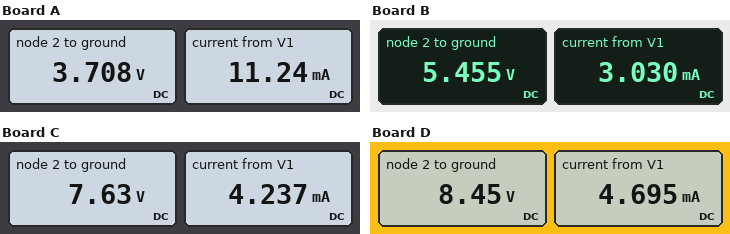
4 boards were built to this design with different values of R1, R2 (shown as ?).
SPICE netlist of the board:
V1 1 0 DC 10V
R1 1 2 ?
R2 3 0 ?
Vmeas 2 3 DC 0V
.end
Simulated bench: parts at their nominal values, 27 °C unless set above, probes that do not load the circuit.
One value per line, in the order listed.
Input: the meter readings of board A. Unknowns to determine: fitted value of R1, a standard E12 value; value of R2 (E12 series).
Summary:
560 Ω
330 Ω
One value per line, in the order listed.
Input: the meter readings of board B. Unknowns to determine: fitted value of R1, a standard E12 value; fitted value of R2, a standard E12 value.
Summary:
1.5 kΩ
1.8 kΩ
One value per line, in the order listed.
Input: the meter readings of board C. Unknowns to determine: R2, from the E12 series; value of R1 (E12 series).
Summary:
1.8 kΩ
560 Ω
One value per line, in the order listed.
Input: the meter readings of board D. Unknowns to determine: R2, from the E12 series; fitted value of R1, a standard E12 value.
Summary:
1.8 kΩ
330 Ω
